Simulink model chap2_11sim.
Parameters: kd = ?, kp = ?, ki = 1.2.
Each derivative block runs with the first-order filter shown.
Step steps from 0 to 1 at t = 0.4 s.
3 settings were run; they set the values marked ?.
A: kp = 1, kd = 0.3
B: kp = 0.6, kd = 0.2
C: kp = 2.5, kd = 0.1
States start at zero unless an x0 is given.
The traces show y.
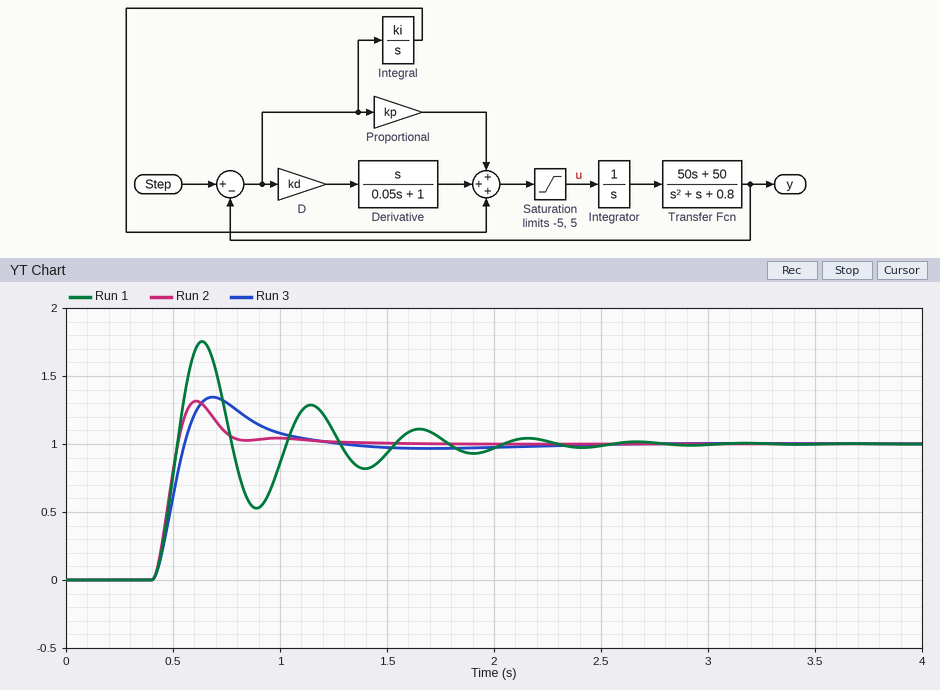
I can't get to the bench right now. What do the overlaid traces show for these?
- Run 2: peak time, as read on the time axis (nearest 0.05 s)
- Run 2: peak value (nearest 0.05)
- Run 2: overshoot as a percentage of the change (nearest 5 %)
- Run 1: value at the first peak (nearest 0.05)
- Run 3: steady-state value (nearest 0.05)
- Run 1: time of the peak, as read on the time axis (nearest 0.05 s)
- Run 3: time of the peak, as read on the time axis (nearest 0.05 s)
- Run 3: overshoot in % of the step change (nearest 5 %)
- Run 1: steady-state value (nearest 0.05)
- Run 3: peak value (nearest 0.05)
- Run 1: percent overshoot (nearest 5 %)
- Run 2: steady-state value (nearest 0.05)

0.60 s
1.30
30 %
1.75
1.00
0.65 s
0.70 s
35 %
1.00
1.35
75 %
1.00
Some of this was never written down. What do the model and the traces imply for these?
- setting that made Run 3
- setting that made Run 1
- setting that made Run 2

B
C
A
